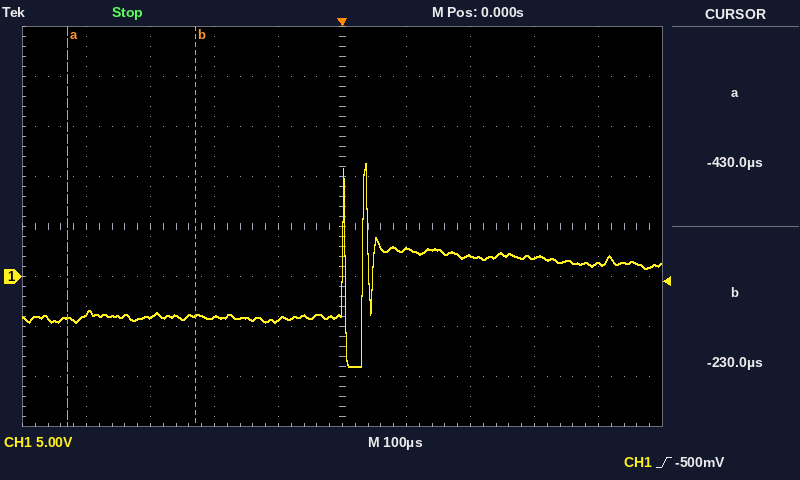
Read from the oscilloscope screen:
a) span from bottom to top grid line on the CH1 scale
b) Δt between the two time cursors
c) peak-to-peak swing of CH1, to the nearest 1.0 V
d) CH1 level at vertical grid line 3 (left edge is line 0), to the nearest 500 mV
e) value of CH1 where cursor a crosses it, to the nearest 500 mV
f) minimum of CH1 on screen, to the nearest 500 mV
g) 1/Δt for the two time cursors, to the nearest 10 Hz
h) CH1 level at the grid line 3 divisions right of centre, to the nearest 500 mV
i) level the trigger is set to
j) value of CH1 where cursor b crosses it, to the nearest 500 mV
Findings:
40 V
200 µs
20.0 V
-4.0 V
-4.0 V
-9.0 V
5.00 kHz
2.0 V
-500 mV
-4.0 V
